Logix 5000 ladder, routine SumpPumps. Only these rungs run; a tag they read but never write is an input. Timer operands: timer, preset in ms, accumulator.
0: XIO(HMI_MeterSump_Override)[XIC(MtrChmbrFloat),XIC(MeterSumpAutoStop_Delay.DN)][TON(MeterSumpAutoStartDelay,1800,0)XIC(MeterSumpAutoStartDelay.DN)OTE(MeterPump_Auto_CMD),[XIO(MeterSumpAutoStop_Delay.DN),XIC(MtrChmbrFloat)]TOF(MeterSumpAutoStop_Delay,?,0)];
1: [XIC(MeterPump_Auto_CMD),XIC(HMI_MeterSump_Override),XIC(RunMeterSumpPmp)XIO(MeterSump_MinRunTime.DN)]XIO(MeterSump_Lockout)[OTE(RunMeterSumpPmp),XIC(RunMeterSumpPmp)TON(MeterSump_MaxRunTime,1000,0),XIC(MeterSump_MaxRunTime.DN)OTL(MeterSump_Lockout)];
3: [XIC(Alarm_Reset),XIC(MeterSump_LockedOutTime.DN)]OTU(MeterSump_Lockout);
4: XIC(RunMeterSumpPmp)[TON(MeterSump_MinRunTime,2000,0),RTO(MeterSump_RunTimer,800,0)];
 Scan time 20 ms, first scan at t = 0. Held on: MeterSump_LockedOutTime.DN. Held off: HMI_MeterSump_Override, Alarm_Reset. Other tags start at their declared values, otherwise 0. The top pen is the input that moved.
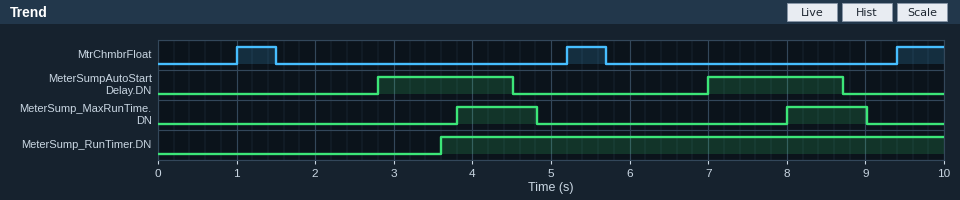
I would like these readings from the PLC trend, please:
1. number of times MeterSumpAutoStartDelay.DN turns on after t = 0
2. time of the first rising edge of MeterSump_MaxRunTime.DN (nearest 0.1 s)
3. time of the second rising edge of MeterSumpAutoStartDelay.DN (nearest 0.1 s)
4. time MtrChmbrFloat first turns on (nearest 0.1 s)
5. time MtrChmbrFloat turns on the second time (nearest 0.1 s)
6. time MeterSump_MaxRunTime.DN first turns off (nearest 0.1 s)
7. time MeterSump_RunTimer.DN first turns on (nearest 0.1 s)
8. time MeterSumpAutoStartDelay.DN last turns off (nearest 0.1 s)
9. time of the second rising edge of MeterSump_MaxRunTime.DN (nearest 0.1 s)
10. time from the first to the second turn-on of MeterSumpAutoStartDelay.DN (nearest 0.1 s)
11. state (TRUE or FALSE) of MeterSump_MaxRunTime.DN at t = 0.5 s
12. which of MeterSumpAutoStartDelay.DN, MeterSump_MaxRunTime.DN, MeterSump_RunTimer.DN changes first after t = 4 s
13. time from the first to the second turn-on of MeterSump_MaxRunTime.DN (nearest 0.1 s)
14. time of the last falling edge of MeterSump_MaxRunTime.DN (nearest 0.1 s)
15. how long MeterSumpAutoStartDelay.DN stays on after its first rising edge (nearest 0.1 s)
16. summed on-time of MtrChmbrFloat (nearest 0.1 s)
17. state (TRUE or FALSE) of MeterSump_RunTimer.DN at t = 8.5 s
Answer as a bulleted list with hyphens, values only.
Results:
- 2
- 3.8 s
- 7.0 s
- 1.0 s
- 5.2 s
- 4.8 s
- 3.6 s
- 8.7 s
- 8.0 s
- 4.2 s
- FALSE
- MeterSumpAutoStartDelay.DN
- 4.2 s
- 9.0 s
- 1.7 s
- 1.6 s
- TRUE
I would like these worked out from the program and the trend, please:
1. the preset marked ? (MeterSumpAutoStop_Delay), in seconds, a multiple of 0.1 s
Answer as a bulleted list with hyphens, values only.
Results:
- 3.0 s
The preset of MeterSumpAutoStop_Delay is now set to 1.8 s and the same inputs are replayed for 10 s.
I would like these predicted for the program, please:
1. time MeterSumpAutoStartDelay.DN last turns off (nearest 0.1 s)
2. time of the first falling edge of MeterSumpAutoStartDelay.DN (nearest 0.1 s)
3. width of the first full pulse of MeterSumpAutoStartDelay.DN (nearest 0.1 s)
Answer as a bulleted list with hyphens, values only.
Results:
- 7.5 s
- 3.3 s
- 0.5 s
